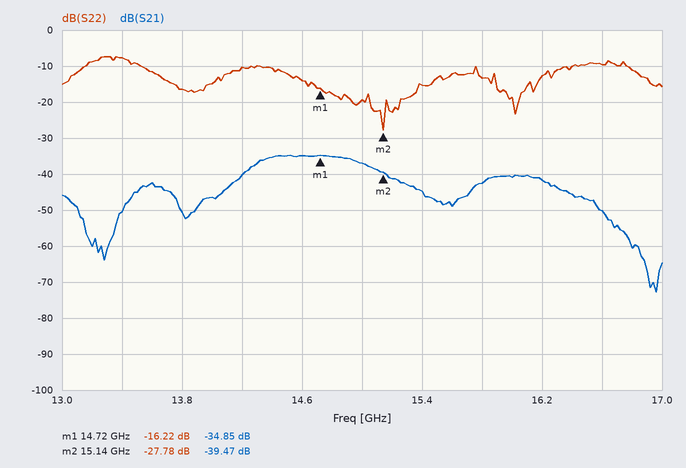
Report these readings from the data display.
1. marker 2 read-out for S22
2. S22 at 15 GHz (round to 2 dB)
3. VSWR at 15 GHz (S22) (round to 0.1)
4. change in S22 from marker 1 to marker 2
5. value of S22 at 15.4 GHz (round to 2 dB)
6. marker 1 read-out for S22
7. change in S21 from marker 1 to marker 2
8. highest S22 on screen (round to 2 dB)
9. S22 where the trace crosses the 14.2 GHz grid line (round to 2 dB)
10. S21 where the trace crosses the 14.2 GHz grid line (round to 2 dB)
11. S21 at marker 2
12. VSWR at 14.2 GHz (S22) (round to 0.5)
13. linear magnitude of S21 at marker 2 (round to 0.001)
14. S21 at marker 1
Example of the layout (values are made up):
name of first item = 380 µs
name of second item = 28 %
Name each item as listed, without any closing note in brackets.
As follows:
marker 2 read-out for S22 = -27.78 dB
S22 at 15 GHz = -20 dB
VSWR at 15 GHz (S22) = 1.2
change in S22 from marker 1 to marker 2 = -11.56 dB
value of S22 at 15.4 GHz = -16 dB
marker 1 read-out for S22 = -16.22 dB
change in S21 from marker 1 to marker 2 = -4.62 dB
highest S22 on screen = -8 dB
S22 where the trace crosses the 14.2 GHz grid line = -10 dB
S21 where the trace crosses the 14.2 GHz grid line = -40 dB
S21 at marker 2 = -39.47 dB
VSWR at 14.2 GHz (S22) = 2.0
linear magnitude of S21 at marker 2 = 0.011
S21 at marker 1 = -34.85 dB
